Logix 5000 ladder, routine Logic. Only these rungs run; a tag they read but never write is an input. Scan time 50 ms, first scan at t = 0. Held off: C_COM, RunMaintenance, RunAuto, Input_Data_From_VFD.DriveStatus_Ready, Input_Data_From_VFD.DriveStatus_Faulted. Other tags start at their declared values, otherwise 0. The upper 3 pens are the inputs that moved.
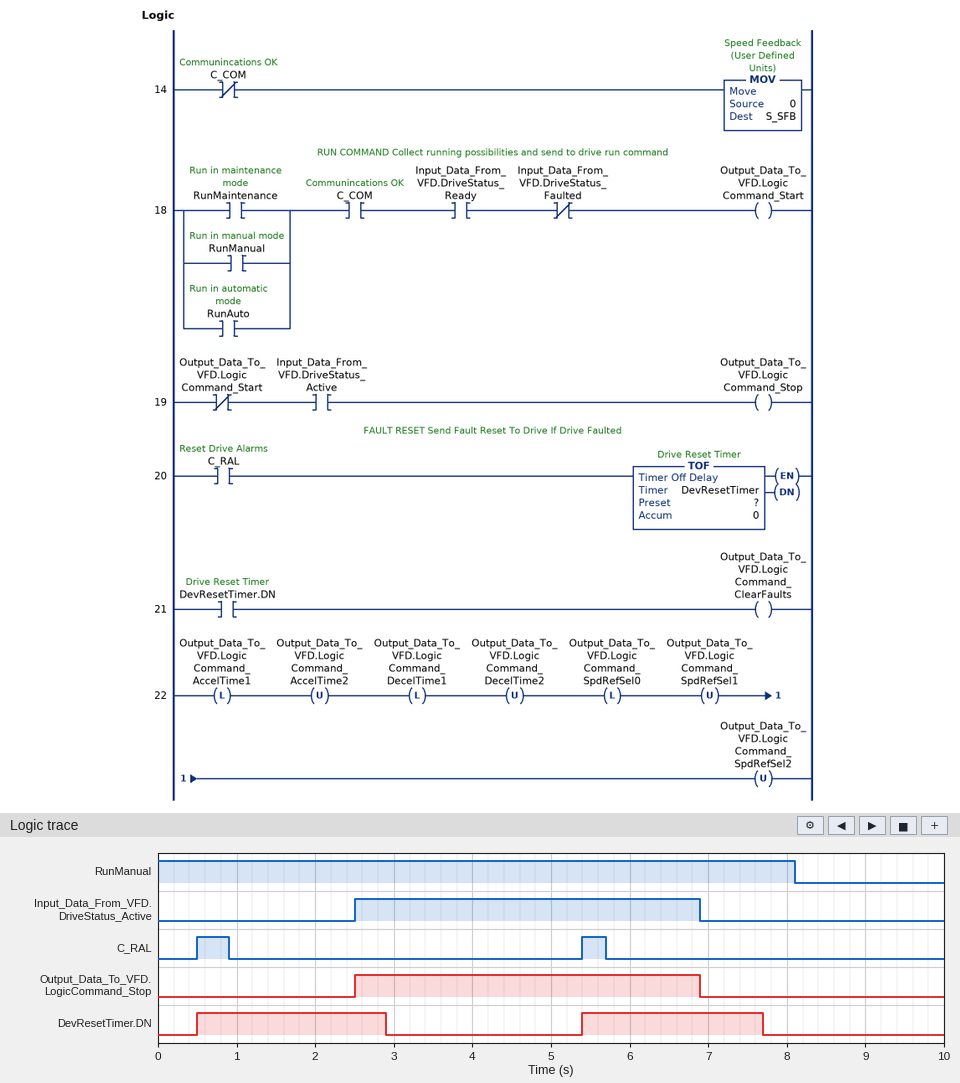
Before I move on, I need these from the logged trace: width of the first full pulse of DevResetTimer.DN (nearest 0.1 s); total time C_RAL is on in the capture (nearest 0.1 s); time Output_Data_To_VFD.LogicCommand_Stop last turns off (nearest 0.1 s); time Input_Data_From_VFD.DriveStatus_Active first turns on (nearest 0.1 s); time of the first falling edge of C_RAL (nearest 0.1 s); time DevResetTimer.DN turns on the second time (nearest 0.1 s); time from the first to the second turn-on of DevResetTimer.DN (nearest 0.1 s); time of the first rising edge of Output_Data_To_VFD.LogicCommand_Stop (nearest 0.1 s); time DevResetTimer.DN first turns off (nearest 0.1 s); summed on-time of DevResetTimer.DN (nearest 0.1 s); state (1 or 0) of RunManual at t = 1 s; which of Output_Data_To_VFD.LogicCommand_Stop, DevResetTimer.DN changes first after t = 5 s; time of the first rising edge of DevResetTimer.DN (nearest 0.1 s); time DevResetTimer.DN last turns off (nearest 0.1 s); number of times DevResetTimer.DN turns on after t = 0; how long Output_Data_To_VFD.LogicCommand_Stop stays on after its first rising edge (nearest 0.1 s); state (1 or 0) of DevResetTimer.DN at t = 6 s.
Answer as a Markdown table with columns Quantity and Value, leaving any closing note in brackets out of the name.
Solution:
| Quantity | Value |
|---|---|
| width of the first full pulse of DevResetTimer.DN | 2.4 s |
| total time C_RAL is on in the capture | 0.7 s |
| time Output_Data_To_VFD.LogicCommand_Stop last turns off | 6.9 s |
| time Input_Data_From_VFD.DriveStatus_Active first turns on | 2.5 s |
| time of the first falling edge of C_RAL | 0.9 s |
| time DevResetTimer.DN turns on the second time | 5.4 s |
| time from the first to the second turn-on of DevResetTimer.DN | 4.9 s |
| time of the first rising edge of Output_Data_To_VFD.LogicCommand_Stop | 2.5 s |
| time DevResetTimer.DN first turns off | 2.9 s |
| summed on-time of DevResetTimer.DN | 4.7 s |
| state (1 or 0) of RunManual at t = 1 s | 1 |
| which of Output_Data_To_VFD.LogicCommand_Stop, DevResetTimer.DN changes first after t = 5 s | DevResetTimer.DN |
| time of the first rising edge of DevResetTimer.DN | 0.5 s |
| time DevResetTimer.DN last turns off | 7.7 s |
| number of times DevResetTimer.DN turns on after t = 0 | 2 |
| how long Output_Data_To_VFD.LogicCommand_Stop stays on after its first rising edge | 4.4 s |
| state (1 or 0) of DevResetTimer.DN at t = 6 s | 1 |
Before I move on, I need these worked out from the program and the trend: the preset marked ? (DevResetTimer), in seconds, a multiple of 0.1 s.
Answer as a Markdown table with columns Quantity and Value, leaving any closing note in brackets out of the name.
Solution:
| Quantity | Value |
|---|---|
| the preset marked ? (DevResetTimer), in seconds, a multiple of 0.1 s | 2.0 s |
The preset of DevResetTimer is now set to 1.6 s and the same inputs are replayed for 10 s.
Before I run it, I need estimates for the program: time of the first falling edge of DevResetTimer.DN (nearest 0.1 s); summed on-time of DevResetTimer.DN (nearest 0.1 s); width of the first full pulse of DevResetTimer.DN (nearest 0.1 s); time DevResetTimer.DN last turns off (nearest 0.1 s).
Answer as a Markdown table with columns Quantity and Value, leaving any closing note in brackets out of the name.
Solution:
| Quantity | Value |
|---|---|
| time of the first falling edge of DevResetTimer.DN | 2.5 s |
| summed on-time of DevResetTimer.DN | 3.9 s |
| width of the first full pulse of DevResetTimer.DN | 2.0 s |
| time DevResetTimer.DN last turns off | 7.3 s |
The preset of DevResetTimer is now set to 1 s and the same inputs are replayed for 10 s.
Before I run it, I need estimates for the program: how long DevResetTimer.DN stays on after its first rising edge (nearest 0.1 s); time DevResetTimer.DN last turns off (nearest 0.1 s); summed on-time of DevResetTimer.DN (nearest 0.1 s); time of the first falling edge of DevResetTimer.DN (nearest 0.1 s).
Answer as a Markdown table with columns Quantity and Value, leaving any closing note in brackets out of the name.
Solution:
| Quantity | Value |
|---|---|
| how long DevResetTimer.DN stays on after its first rising edge | 1.4 s |
| time DevResetTimer.DN last turns off | 6.7 s |
| summed on-time of DevResetTimer.DN | 2.7 s |
| time of the first falling edge of DevResetTimer.DN | 1.9 s |
